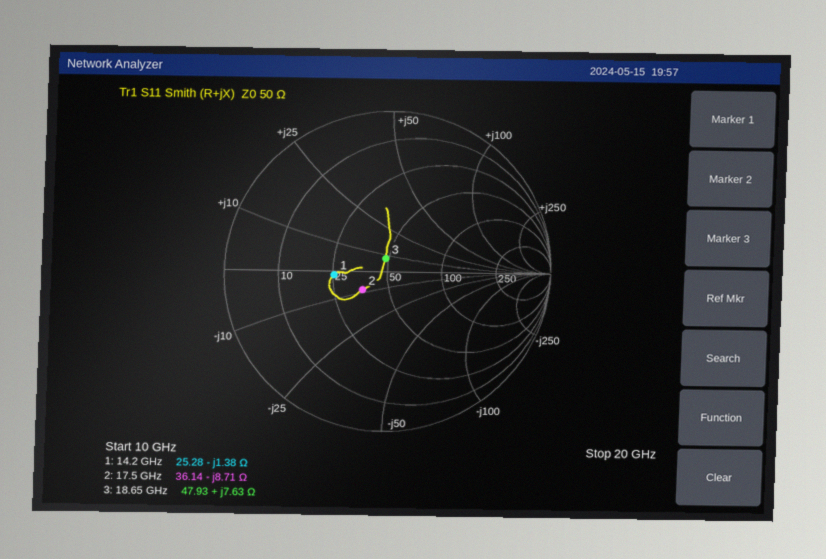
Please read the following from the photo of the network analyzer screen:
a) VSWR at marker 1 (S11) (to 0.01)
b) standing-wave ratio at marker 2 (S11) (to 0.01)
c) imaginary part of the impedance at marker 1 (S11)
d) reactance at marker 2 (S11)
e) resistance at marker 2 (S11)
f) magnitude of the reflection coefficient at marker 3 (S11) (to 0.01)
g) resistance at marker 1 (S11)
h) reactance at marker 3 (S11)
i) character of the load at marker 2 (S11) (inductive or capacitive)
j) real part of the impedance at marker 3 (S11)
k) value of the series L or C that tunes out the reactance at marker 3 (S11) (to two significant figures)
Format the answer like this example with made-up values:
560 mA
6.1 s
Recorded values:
1.98
1.47
-1.38 Ω
-8.71 Ω
36.14 Ω
0.08
25.28 Ω
+7.63 Ω
capacitive
47.93 Ω
1.1 pF
